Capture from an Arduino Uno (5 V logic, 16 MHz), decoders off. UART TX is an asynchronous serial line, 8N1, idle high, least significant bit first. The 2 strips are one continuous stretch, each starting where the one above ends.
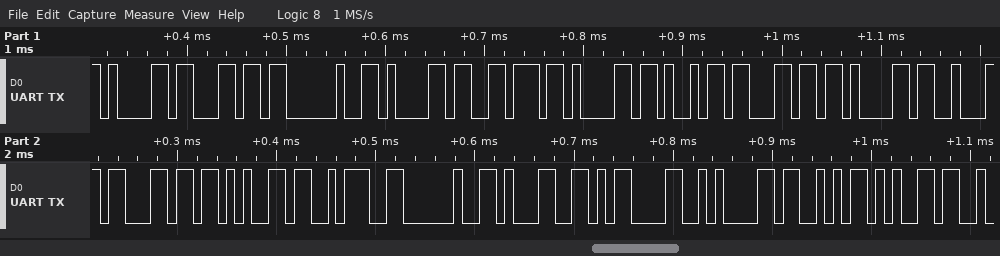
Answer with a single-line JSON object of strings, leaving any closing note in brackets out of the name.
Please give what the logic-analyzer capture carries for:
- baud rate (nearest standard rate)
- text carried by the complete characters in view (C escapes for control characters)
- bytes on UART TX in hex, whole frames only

{"baud rate": "115200 baud", "text carried by the complete characters in view": "\"al available: 1\\r\\nSe\"", "bytes on UART TX in hex, whole frames only": "61 6C 20 61 76 61 69 6C 61 62 6C 65 3A 20 31 0D 0A 53 65"}
